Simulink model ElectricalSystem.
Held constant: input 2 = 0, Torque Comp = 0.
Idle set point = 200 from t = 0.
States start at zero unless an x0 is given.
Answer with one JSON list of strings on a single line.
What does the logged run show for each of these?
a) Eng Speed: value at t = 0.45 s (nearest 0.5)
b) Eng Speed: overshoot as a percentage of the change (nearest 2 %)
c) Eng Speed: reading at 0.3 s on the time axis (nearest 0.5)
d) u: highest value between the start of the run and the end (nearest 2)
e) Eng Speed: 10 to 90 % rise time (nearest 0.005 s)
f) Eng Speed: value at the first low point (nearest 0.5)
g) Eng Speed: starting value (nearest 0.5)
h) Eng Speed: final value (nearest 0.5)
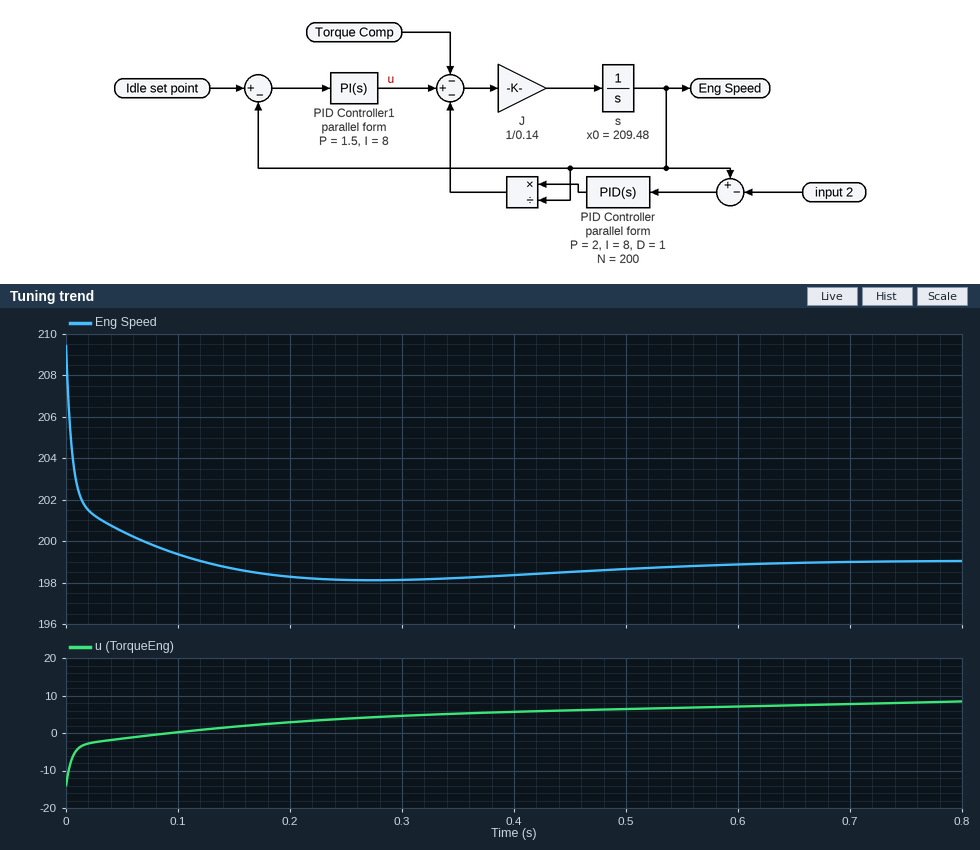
["198.5", "8 %", "198.0", "8", "0.065 s", "198.0", "209.5", "199.0"]
